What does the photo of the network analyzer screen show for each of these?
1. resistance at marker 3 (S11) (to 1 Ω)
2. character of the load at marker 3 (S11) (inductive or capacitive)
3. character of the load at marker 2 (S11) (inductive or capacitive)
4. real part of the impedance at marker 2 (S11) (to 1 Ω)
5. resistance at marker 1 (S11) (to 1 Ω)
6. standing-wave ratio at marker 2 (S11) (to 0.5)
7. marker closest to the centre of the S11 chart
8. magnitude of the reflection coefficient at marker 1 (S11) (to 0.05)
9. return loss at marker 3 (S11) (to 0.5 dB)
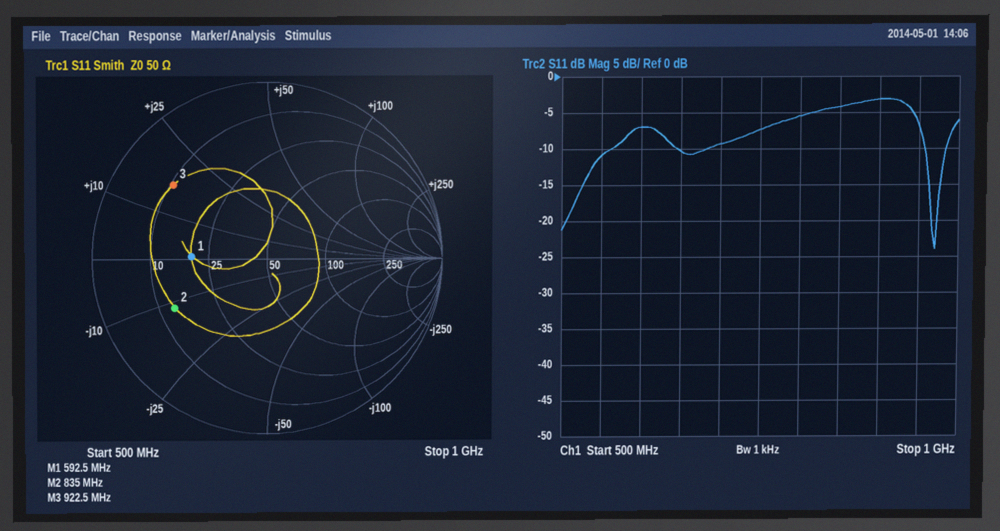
11 Ω
inductive
capacitive
13 Ω
20 Ω
4.0
marker 1
0.45
3.5 dB
